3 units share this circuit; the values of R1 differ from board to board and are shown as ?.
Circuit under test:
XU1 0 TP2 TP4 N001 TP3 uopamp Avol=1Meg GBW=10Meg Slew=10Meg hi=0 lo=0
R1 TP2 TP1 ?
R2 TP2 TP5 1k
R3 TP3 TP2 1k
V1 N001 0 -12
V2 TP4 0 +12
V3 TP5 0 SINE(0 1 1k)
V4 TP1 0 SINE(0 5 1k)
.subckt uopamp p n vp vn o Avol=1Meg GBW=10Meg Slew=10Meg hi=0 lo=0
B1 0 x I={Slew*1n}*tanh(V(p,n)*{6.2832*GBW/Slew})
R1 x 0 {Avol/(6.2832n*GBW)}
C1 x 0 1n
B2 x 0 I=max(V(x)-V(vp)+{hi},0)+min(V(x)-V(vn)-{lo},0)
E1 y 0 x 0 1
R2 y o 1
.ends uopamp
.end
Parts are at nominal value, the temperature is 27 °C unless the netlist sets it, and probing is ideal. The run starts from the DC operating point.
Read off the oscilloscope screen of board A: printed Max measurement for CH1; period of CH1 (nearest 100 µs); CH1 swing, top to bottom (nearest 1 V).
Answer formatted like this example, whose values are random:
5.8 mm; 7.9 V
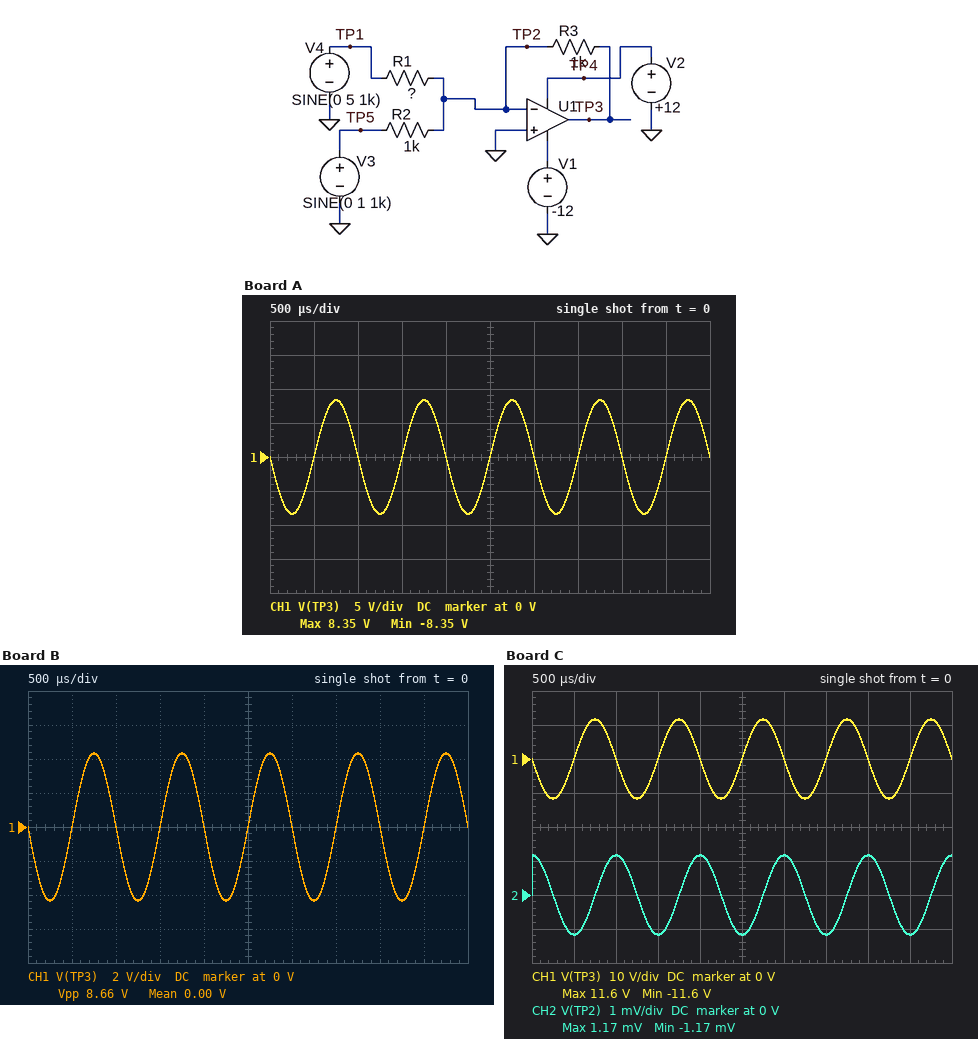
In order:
8.35 V; 1.0 ms; 17 V
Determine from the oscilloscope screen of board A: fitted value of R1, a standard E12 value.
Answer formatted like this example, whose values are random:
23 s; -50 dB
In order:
680 Ω
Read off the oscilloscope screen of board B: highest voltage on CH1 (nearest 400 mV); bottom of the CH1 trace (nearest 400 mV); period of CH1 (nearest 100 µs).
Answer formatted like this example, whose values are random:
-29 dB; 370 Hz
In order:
4.4 V; -4.4 V; 1.0 ms
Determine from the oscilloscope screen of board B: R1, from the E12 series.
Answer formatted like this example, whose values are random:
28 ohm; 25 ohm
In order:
1.5 kΩ
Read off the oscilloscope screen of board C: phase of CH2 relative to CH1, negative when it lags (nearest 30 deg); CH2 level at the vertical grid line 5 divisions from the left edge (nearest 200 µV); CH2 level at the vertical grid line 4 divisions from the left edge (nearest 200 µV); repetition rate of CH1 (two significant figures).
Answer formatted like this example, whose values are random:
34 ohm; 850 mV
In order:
-90 deg; -1.2 mV; 1.2 mV; 1.0 kHz
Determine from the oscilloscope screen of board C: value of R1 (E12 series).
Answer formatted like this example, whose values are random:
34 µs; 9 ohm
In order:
470 Ω
